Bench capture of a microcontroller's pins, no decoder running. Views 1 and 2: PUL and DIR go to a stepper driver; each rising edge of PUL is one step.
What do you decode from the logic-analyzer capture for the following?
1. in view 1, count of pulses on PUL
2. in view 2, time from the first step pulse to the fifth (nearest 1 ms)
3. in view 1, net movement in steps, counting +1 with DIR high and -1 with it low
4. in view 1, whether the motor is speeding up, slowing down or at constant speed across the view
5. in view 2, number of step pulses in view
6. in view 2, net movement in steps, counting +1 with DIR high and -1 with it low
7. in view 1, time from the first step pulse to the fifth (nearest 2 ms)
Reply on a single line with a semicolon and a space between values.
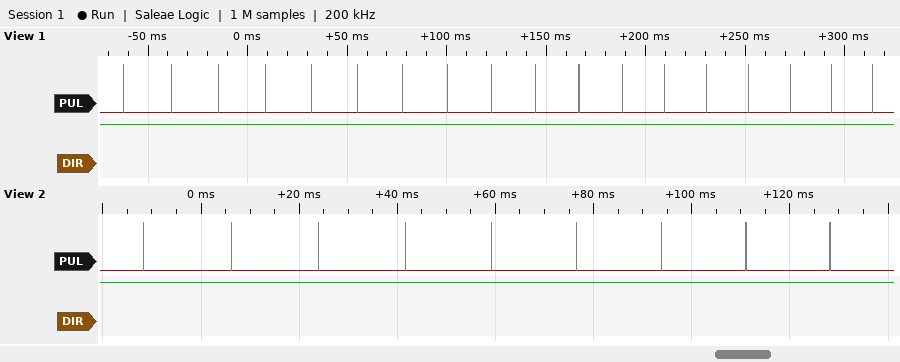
18; 71 ms; +18; speeding up; 9; +9; 94 ms
